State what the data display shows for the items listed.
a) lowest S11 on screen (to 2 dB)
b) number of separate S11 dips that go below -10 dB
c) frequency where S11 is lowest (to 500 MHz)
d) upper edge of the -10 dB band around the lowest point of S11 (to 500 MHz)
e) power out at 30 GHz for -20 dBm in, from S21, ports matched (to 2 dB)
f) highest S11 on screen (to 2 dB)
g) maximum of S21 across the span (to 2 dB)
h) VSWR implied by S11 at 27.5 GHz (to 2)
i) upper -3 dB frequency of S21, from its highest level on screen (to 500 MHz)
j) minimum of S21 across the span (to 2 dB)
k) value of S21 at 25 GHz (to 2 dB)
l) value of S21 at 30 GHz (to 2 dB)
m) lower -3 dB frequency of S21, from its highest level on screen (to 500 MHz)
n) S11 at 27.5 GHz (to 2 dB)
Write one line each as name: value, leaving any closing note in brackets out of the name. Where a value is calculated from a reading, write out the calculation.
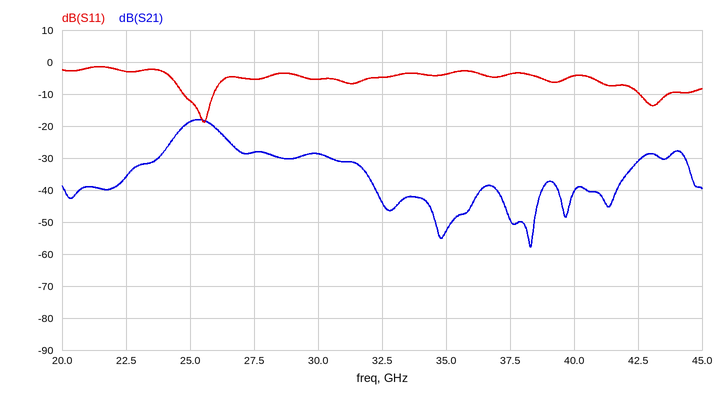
lowest S11 on screen: -18 dB
number of separate S11 dips that go below -10 dB: 2
frequency where S11 is lowest: 25.5 GHz
upper edge of the -10 dB band around the lowest point of S11: 26.0 GHz
power out at 30 GHz for -20 dBm in, from S21, ports matched: -20 dBm + (-28 dB) = -48 dBm
highest S11 on screen: -2 dB
maximum of S21 across the span: -18 dB
VSWR implied by S11 at 27.5 GHz: |Γ| = 10^(-6/20) = 0.5012; VSWR = (1 + 0.5012)/(1 − 0.5012) ≈ 3.01, so 4 to the nearest 2
upper -3 dB frequency of S21, from its highest level on screen: 26.0 GHz
minimum of S21 across the span: -58 dB
value of S21 at 25 GHz: -18 dB
value of S21 at 30 GHz: -28 dB
lower -3 dB frequency of S21, from its highest level on screen: 24.5 GHz
S11 at 27.5 GHz: -6 dB
